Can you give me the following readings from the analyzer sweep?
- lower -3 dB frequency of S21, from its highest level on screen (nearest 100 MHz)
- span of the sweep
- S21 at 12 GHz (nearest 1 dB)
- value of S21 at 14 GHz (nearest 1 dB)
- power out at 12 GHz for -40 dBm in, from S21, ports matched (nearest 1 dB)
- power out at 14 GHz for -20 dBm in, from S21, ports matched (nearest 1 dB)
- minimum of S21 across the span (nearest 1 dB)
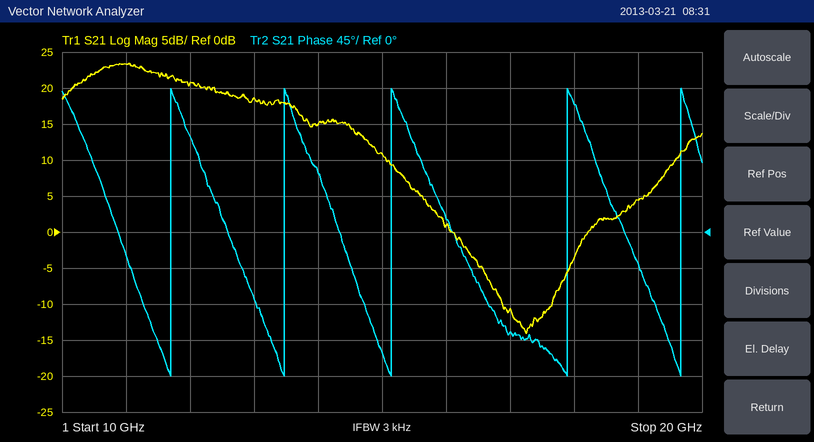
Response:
10.2 GHz
10 GHz
21 dB
15 dB
-19 dBm
-5 dBm
-14 dB
